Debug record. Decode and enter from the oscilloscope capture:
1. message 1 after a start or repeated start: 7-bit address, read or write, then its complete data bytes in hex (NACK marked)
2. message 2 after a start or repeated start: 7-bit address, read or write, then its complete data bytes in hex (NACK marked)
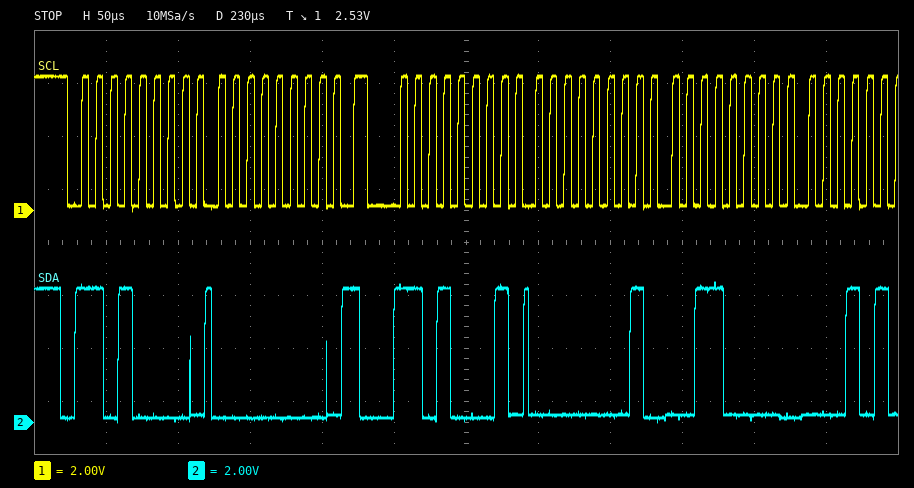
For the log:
0x68 write: 00
0x68 read: 01 30
